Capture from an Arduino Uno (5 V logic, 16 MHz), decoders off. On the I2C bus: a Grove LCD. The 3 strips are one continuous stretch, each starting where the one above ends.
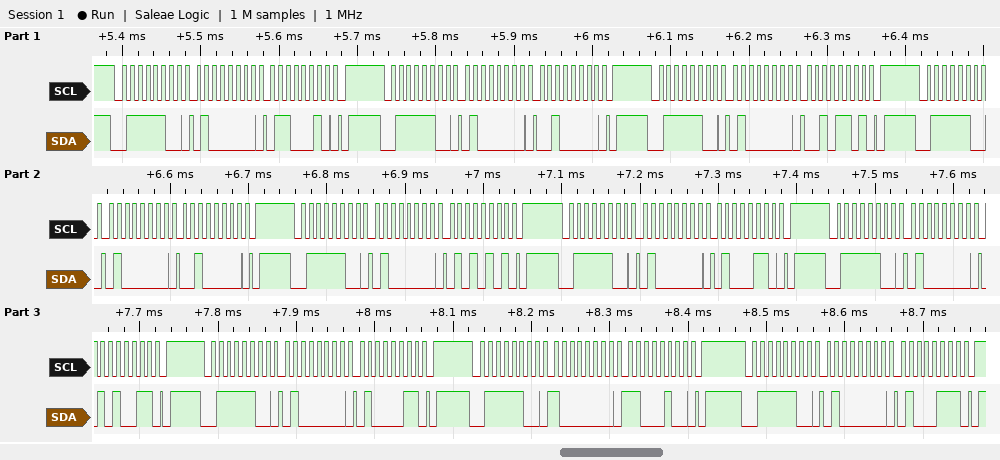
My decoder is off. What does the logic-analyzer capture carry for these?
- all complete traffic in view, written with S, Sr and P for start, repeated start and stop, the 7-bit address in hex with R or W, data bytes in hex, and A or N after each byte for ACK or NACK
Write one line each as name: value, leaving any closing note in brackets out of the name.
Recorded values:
all complete traffic in view, written with S, Sr and P for start, repeated start and stop, the 7-bit address in hex with R or W, data bytes in hex, and A or N after each byte for ACK or NACK: S 3EW A 40 A 62 A P S 3EW A 40 A 20 A P S 3EW A 40 A 2D A P S 3EW A 40 A 20 A P S 3EW A 40 A 55 A P S 3EW A 40 A 46 A P S 3EW A 40 A 53 A P S 3EW A 40 A 43 A P S 3EW A 80 A C4 A P S 3EW A 40 A 47 A P
